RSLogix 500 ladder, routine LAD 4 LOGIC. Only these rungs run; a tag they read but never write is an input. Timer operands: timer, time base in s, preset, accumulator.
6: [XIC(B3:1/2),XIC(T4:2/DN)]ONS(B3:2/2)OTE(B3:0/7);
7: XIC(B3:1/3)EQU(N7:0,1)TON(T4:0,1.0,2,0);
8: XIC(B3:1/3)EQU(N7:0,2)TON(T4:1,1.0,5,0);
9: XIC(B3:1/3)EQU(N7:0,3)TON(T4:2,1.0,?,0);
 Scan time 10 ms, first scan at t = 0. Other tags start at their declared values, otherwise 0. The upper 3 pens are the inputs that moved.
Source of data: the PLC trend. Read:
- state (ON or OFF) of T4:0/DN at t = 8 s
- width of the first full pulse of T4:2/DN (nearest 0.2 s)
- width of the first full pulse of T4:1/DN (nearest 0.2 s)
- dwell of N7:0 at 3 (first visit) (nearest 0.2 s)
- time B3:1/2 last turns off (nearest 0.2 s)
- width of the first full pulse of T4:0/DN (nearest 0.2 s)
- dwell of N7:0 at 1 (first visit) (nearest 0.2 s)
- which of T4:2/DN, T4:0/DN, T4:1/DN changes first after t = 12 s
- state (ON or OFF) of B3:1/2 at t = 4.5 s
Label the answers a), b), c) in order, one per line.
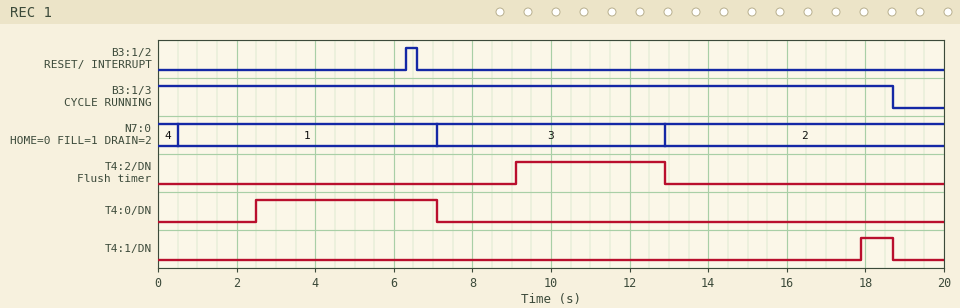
a) OFF
b) 3.8 s
c) 0.8 s
d) 5.8 s
e) 6.6 s
f) 4.6 s
g) 6.6 s
h) T4:2/DN
i) OFF
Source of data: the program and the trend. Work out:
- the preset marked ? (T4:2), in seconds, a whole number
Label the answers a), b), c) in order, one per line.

a) 2 s
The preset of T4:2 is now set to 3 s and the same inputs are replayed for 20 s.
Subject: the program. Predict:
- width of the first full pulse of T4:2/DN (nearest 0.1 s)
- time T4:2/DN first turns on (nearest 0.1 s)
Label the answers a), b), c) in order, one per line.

a) 2.8 s
b) 10.1 s
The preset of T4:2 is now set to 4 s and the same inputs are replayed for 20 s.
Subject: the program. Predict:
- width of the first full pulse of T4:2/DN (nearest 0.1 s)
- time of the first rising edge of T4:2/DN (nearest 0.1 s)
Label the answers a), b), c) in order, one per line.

a) 1.8 s
b) 11.1 s
